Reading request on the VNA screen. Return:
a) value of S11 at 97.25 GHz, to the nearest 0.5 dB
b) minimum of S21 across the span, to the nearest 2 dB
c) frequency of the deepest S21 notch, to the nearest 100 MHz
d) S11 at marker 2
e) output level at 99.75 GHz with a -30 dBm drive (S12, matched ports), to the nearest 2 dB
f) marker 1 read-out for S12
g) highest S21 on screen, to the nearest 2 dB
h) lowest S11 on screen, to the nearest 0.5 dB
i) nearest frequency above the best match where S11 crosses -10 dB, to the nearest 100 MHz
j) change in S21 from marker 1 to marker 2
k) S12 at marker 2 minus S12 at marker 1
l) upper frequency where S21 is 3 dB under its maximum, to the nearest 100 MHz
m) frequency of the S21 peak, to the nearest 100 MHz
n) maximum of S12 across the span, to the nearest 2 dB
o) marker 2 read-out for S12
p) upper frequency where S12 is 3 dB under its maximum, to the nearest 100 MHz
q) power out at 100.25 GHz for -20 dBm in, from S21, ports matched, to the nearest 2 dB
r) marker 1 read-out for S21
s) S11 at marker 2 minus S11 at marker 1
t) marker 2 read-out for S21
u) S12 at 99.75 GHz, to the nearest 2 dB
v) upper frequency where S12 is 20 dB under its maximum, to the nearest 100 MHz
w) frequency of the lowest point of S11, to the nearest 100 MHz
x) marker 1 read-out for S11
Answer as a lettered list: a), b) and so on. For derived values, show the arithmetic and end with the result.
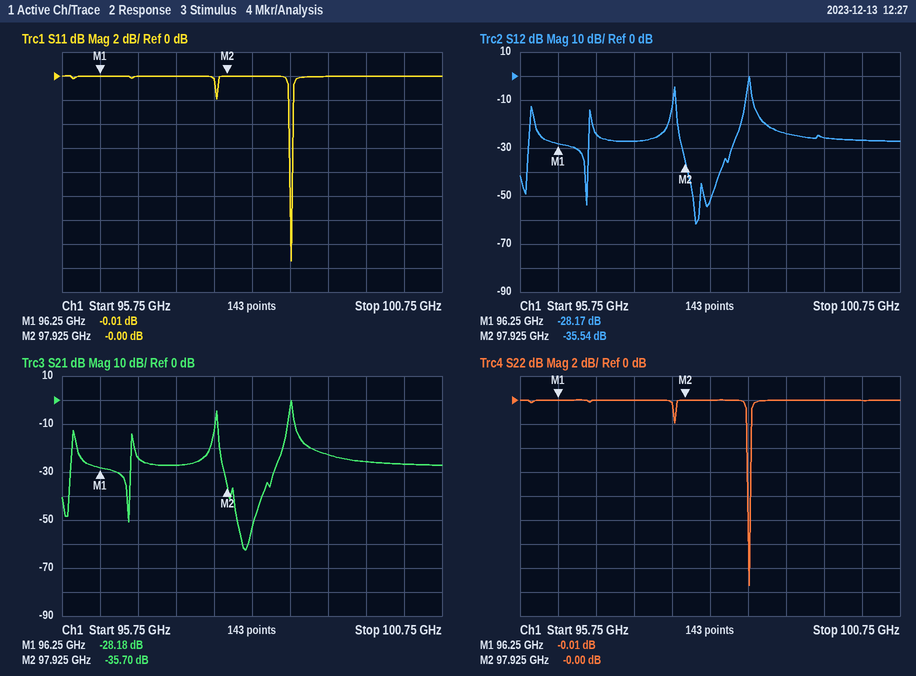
a) 0.0 dB
b) -62 dB
c) 98.2 GHz
d) -0.00 dB
e) -30 dBm + (-26 dB) = -56 dBm
f) -28.17 dB
g) 0 dB
h) -15.5 dB
i) 98.8 GHz
j) -35.7 − (-28.18) = -7.52 dB
k) -35.54 − (-28.17) = -7.37 dB
l) 98.8 GHz
m) 98.8 GHz
n) 0 dB
o) -35.54 dB
p) 98.8 GHz
q) -20 dBm + (-26 dB) = -46 dBm
r) -28.18 dB
s) -0 − (-0.01) = 0.01 dB
t) -35.70 dB
u) -26 dB
v) 99.0 GHz
w) 98.8 GHz
x) -0.01 dB
